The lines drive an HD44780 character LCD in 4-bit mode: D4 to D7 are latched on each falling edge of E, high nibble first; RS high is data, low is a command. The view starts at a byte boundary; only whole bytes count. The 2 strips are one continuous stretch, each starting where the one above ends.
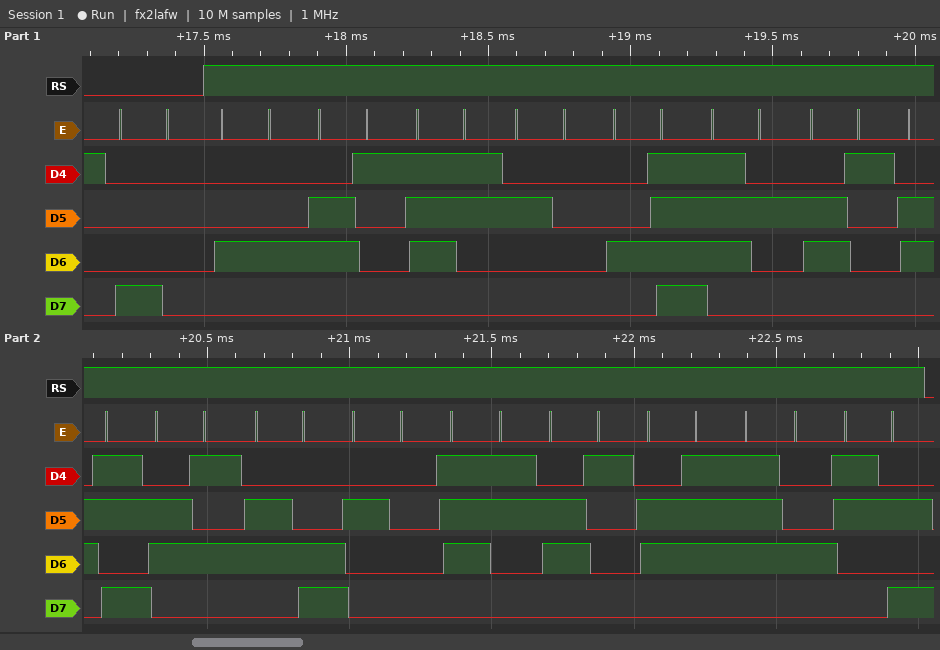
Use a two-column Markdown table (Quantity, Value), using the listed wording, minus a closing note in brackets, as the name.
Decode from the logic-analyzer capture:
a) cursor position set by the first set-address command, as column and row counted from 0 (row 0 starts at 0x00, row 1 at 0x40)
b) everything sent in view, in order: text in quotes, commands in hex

| Quantity | Value |
|---|---|
| cursor position set by the first set-address command, as column and row counted from 0 | column 0, row 0 |
| everything sent in view, in order: text in quotes, commands in hex | 0x80 "Das Orakel sagt:" |
